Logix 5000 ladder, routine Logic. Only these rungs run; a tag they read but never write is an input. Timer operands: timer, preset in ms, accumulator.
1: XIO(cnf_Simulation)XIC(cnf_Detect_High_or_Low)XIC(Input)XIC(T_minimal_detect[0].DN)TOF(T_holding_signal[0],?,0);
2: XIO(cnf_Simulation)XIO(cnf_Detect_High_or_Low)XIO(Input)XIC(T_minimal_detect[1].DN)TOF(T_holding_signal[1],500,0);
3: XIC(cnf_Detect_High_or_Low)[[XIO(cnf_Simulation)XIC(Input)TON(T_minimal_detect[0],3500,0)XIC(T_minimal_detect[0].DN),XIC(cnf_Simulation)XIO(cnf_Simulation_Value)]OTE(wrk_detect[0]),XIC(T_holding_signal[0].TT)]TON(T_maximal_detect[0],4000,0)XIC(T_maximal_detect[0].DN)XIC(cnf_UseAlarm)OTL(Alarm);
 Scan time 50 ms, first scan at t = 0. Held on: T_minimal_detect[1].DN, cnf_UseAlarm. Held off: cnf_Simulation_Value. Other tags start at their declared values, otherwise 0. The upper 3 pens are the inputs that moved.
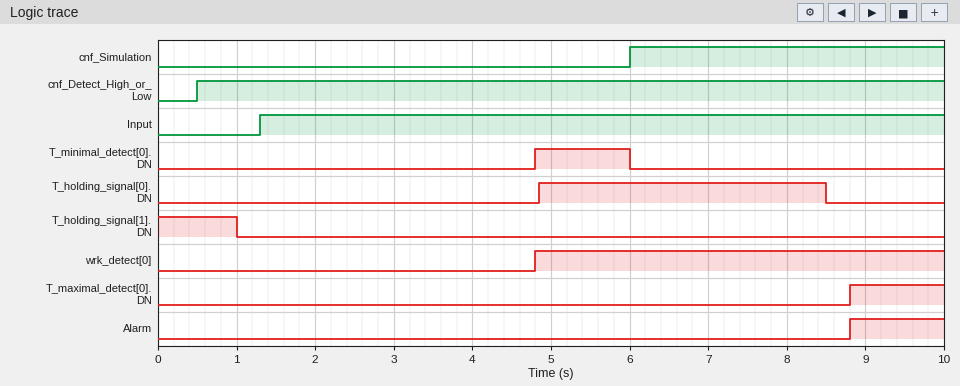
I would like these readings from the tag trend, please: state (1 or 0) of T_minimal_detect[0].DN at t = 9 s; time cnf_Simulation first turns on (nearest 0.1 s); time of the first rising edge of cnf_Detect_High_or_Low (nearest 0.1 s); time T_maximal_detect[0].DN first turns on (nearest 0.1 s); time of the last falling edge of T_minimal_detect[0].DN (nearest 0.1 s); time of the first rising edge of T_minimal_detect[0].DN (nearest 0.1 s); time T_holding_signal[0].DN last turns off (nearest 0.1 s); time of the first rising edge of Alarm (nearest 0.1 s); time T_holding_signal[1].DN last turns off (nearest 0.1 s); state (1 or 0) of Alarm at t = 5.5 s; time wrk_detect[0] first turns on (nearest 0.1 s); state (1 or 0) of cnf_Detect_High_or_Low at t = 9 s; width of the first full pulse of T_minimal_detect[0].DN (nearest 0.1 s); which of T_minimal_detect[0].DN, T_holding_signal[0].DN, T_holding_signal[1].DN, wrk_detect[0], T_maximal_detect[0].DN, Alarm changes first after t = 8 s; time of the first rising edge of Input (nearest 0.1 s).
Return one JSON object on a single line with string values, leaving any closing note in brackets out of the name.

{"state (1 or 0) of T_minimal_detect[0].DN at t = 9 s": "0", "time cnf_Simulation first turns on": "6.0 s", "time of the first rising edge of cnf_Detect_High_or_Low": "0.5 s", "time T_maximal_detect[0].DN first turns on": "8.8 s", "time of the last falling edge of T_minimal_detect[0].DN": "6.0 s", "time of the first rising edge of T_minimal_detect[0].DN": "4.8 s", "time T_holding_signal[0].DN last turns off": "8.5 s", "time of the first rising edge of Alarm": "8.8 s", "time T_holding_signal[1].DN last turns off": "1.0 s", "state (1 or 0) of Alarm at t = 5.5 s": "0", "time wrk_detect[0] first turns on": "4.8 s", "state (1 or 0) of cnf_Detect_High_or_Low at t = 9 s": "1", "width of the first full pulse of T_minimal_detect[0].DN": "1.2 s", "which of T_minimal_detect[0].DN, T_holding_signal[0].DN, T_holding_signal[1].DN, wrk_detect[0], T_maximal_detect[0].DN, Alarm changes first after t = 8 s": "T_holding_signal[0].DN", "time of the first rising edge of Input": "1.3 s"}
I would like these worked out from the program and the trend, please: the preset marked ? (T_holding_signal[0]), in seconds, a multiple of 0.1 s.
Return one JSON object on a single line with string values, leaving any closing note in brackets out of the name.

{"the preset marked ? (T_holding_signal[0]), in seconds, a multiple of 0.1 s": "2.5 s"}
